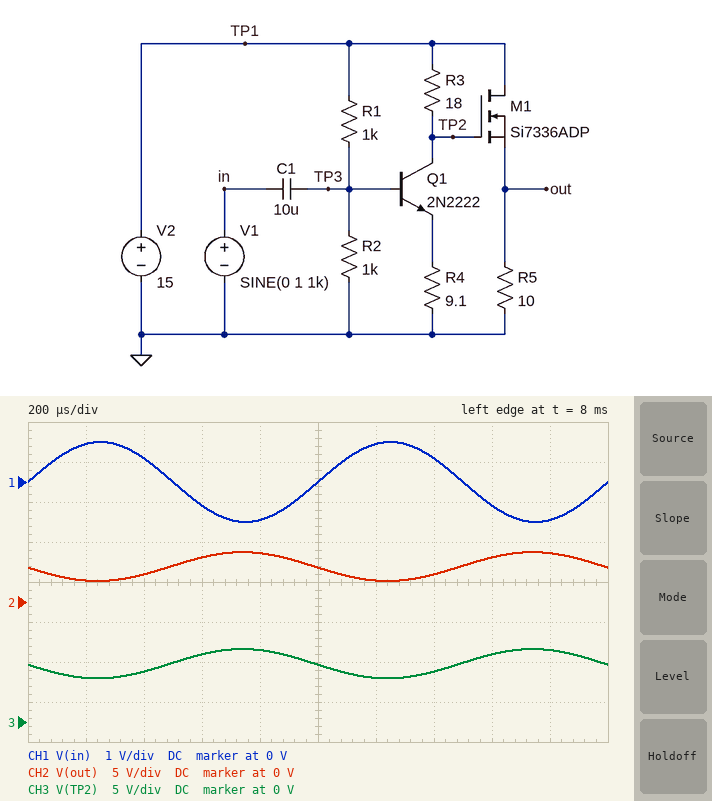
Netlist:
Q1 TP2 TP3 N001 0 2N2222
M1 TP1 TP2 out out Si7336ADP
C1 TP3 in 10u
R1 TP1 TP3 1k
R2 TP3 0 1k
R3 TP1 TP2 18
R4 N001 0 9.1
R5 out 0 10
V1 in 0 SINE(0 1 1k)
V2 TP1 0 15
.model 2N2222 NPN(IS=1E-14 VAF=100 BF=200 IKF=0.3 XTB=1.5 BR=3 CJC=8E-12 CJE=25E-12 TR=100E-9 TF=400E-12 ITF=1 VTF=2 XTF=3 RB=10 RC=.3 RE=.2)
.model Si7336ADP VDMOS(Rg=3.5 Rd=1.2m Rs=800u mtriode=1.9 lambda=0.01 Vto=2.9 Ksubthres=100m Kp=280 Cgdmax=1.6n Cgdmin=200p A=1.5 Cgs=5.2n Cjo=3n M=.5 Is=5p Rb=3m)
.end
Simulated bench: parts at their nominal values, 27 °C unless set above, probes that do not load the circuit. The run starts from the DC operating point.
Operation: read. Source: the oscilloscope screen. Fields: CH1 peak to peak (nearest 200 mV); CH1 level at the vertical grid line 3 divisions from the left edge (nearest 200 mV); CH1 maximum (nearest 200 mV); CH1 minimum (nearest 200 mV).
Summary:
2.0 V
-600 mV
1.0 V
-1.0 V
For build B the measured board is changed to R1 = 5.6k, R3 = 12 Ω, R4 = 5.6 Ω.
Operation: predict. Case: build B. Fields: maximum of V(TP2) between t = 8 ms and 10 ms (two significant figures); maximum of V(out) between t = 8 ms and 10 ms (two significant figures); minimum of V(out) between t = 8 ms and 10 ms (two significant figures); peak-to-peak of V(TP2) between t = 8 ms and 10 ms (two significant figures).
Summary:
15 V
12 V
8.7 V
3.4 V
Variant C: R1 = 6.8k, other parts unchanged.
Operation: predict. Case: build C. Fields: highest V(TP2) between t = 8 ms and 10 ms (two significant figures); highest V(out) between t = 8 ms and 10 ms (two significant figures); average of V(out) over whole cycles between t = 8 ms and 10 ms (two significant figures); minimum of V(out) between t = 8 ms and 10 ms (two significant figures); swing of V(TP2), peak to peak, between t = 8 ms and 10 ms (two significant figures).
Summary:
15 V
12 V
11 V
8.9 V
3.2 V
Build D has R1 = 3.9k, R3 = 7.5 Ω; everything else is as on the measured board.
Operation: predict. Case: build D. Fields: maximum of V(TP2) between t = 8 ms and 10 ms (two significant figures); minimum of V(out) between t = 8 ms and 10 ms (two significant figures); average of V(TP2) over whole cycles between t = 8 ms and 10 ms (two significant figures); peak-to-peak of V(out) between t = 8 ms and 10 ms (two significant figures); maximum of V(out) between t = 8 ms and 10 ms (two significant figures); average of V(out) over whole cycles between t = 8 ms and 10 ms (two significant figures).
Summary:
15 V
10 V
14 V
1.5 V
12 V
11 V
